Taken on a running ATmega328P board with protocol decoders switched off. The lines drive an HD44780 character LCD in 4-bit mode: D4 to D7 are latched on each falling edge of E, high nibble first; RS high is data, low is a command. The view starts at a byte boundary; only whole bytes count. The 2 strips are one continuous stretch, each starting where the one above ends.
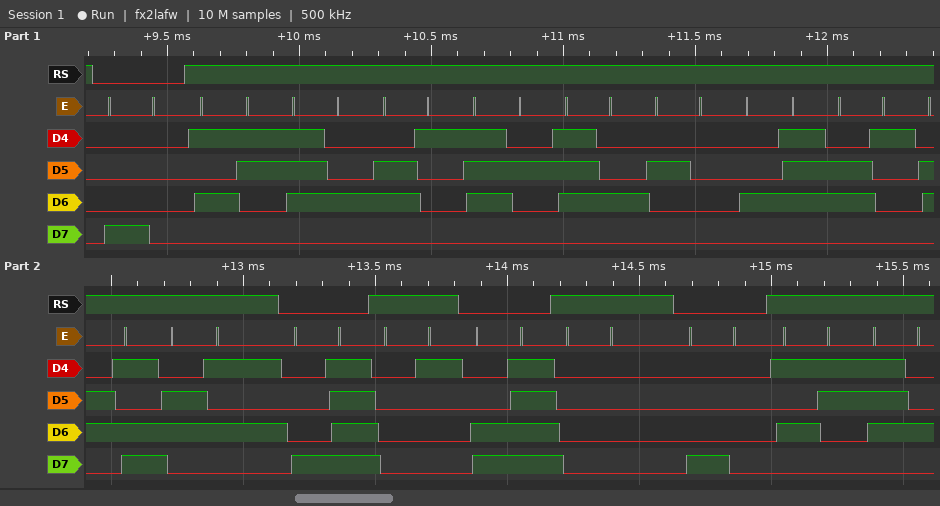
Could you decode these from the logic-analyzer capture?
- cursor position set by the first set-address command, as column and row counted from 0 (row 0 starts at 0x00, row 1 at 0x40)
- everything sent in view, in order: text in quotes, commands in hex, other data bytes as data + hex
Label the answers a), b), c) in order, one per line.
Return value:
a) column 0, row 0
b) 0x80 "Start Game" 0x8F data 01 0xCF data 00 0x80 "St"
